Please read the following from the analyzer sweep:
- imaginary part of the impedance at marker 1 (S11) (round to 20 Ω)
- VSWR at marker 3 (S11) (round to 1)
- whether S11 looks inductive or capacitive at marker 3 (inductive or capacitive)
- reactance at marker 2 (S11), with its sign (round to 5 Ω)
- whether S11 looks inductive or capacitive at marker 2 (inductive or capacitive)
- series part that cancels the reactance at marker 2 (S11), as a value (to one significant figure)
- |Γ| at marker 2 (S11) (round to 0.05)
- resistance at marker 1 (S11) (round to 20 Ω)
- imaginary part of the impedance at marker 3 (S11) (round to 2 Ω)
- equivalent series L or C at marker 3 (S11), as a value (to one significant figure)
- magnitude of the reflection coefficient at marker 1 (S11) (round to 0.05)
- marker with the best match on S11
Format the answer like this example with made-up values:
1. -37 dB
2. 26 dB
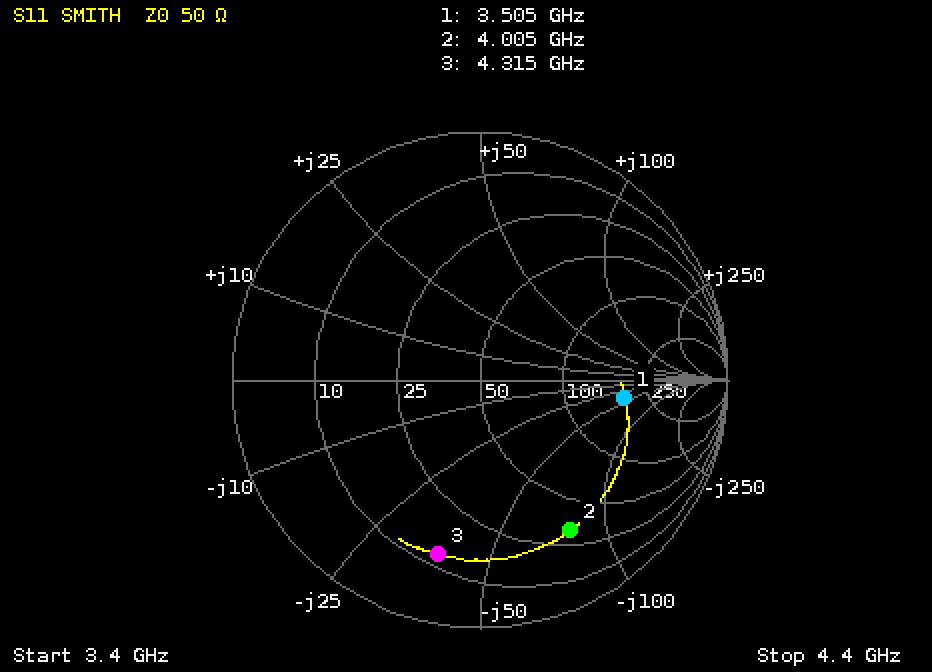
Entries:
1. -40 Ω
2. 6
3. capacitive
4. -80 Ω
5. capacitive
6. 3 nH
7. 0.70
8. 180 Ω
9. -38 Ω
10. 1.0 pF
11. 0.60
12. marker 1
